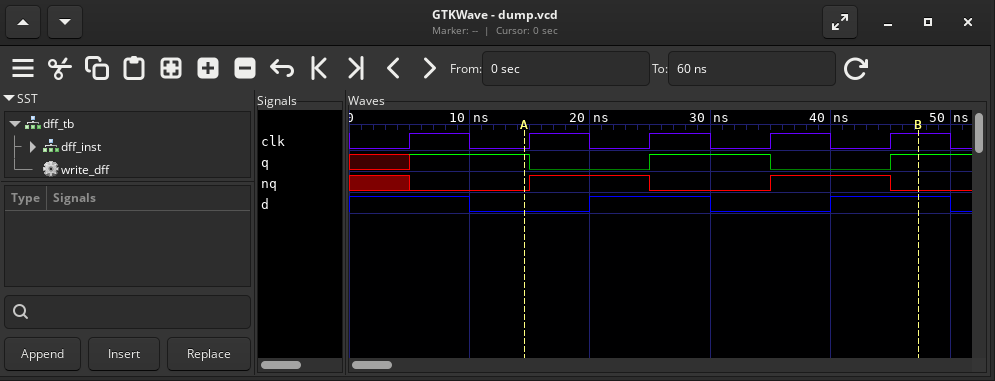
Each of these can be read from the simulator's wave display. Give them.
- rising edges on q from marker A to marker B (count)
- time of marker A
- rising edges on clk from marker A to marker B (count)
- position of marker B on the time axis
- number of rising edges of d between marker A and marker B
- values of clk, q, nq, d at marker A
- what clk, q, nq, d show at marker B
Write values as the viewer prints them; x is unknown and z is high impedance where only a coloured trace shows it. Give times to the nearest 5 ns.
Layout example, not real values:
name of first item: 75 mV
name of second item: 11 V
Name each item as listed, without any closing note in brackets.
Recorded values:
rising edges on q from marker A to marker B: 2
time of marker A: 15 ns
rising edges on clk from marker A to marker B: 4
position of marker B on the time axis: 45 ns
number of rising edges of d between marker A and marker B: 2
values of clk, q, nq, d at marker A: clk=0, q=1, nq=0, d=0
what clk, q, nq, d show at marker B: clk=1, q=1, nq=0, d=1
